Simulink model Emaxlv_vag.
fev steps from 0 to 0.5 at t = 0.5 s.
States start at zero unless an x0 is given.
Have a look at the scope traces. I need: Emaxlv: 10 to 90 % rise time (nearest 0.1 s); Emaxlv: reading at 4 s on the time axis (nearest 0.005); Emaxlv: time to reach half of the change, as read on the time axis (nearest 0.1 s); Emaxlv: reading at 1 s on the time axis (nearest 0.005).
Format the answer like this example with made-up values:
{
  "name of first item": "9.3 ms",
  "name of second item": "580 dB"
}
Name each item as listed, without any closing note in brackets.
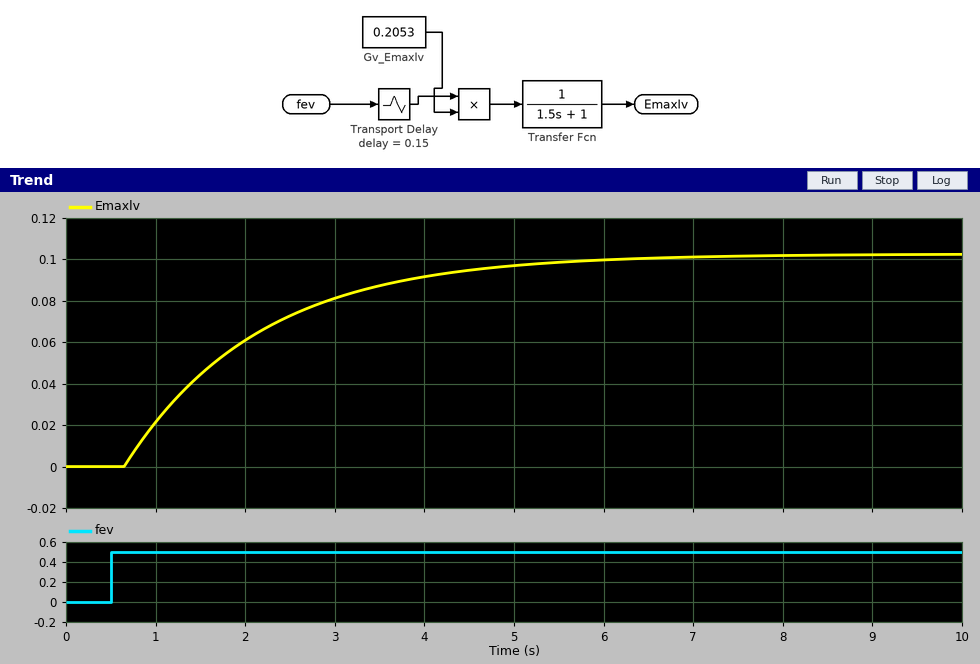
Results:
{
  "Emaxlv: 10 to 90 % rise time": "3.3 s",
  "Emaxlv: reading at 4 s on the time axis": "0.090",
  "Emaxlv: time to reach half of the change, as read on the time axis": "1.7 s",
  "Emaxlv: reading at 1 s on the time axis": "0.020"
}
